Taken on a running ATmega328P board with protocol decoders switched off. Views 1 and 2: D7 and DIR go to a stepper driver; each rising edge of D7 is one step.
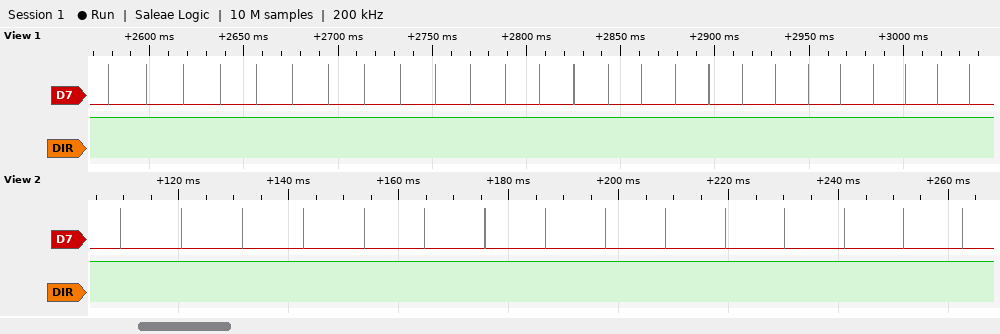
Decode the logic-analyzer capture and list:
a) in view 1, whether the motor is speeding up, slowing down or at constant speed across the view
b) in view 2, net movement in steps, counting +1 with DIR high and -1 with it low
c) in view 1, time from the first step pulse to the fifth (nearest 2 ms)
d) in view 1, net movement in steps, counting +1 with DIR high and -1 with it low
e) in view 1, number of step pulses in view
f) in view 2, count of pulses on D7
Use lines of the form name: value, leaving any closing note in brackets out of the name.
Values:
in view 1, whether the motor is speeding up, slowing down or at constant speed across the view: speeding up
in view 2, net movement in steps, counting +1 with DIR high and -1 with it low: +15
in view 1, time from the first step pulse to the fifth: 78 ms
in view 1, net movement in steps, counting +1 with DIR high and -1 with it low: +26
in view 1, number of step pulses in view: 26
in view 2, count of pulses on D7: 15
